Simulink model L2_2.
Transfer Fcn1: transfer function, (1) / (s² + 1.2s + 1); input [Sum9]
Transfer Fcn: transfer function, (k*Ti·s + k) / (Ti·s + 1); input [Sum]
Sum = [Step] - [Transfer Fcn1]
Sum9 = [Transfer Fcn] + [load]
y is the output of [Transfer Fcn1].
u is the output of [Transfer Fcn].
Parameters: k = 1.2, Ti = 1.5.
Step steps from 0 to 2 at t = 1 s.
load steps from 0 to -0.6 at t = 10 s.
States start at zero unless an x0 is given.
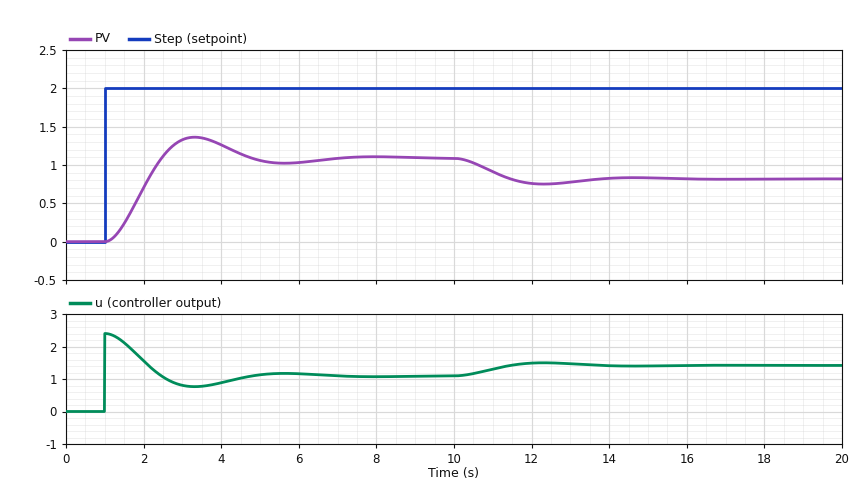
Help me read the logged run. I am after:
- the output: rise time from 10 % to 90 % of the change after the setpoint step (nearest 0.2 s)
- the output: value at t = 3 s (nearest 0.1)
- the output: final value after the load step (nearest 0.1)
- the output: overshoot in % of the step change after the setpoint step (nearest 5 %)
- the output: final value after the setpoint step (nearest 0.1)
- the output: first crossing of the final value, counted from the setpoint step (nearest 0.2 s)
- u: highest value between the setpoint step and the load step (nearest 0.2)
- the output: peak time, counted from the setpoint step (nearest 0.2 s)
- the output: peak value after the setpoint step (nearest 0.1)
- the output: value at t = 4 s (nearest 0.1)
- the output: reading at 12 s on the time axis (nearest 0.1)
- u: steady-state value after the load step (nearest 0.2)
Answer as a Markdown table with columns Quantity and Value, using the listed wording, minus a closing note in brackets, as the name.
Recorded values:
| Quantity | Value |
|---|---|
| the output: rise time from 10 % to 90 % of the change after the setpoint step | 1.0 s |
| the output: value at t = 3 s | 1.3 |
| the output: final value after the load step | 0.8 |
| the output: overshoot in % of the step change after the setpoint step | 25 % |
| the output: final value after the setpoint step | 1.1 |
| the output: first crossing of the final value, counted from the setpoint step | 1.4 s |
| u: highest value between the setpoint step and the load step | 2.4 |
| the output: peak time, counted from the setpoint step | 2.4 s |
| the output: peak value after the setpoint step | 1.4 |
| the output: value at t = 4 s | 1.3 |
| the output: reading at 12 s on the time axis | 0.8 |
| u: steady-state value after the load step | 1.4 |
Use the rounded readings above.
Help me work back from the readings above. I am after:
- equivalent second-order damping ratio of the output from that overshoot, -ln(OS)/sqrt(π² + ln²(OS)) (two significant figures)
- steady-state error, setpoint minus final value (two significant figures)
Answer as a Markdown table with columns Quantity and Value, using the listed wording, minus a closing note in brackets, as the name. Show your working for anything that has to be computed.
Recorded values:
| Quantity | Value |
|---|---|
| equivalent second-order damping ratio of the output from that overshoot, -ln(OS)/sqrt(π² + ln²(OS)) | ln(0.25) = -1.386; 1.386 / sqrt(9.870 + 1.922) = 0.40 |
| steady-state error, setpoint minus final value | 2 - 1.1 = 0.90 |
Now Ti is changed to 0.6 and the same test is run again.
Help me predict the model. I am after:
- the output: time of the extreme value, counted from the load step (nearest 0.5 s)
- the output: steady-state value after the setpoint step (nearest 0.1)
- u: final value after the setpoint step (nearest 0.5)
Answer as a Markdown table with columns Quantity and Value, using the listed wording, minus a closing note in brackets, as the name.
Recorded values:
| Quantity | Value |
|---|---|
| the output: time of the extreme value, counted from the load step | 2.5 s |
| the output: steady-state value after the setpoint step | 1.1 |
| u: final value after the setpoint step | 1.0 |
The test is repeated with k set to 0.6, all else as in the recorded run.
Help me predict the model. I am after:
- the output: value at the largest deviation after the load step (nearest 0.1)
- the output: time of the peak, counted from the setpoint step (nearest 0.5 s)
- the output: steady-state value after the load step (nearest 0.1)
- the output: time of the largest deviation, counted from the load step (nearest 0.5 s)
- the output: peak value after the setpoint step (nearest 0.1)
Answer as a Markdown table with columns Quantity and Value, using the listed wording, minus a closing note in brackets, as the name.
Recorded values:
| Quantity | Value |
|---|---|
| the output: value at the largest deviation after the load step | 0.3 |
| the output: time of the peak, counted from the setpoint step | 3.0 s |
| the output: steady-state value after the load step | 0.4 |
| the output: time of the largest deviation, counted from the load step | 3.0 s |
| the output: peak value after the setpoint step | 0.9 |
